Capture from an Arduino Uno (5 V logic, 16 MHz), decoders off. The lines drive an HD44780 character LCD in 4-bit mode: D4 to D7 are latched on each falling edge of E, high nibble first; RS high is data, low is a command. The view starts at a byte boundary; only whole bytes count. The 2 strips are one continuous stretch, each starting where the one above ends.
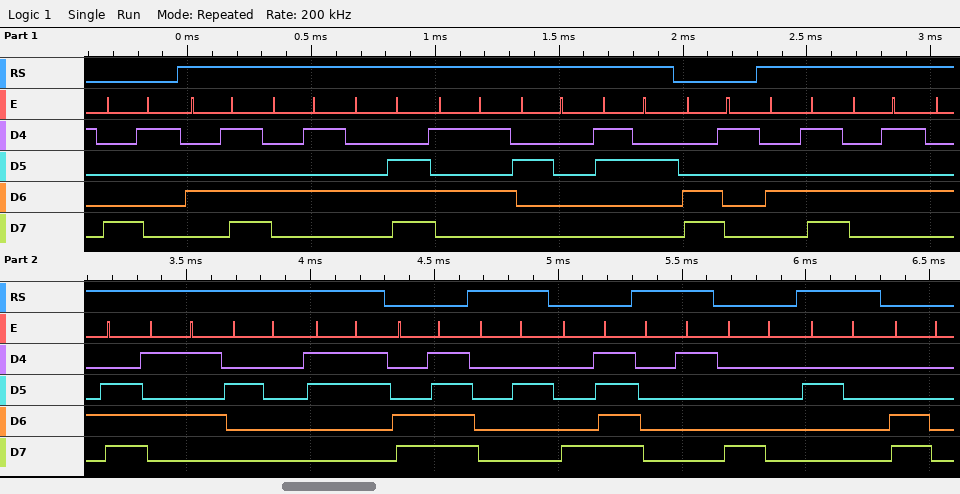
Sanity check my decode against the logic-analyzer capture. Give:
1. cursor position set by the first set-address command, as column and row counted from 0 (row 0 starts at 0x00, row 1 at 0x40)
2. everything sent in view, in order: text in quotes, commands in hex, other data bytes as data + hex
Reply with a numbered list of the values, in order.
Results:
1. column 1, row 0
2. 0x81 "MENU 2" 0xC1 "MENU 3" 0xCF data 02 0x8F data 01 0x80 " " 0xC0
